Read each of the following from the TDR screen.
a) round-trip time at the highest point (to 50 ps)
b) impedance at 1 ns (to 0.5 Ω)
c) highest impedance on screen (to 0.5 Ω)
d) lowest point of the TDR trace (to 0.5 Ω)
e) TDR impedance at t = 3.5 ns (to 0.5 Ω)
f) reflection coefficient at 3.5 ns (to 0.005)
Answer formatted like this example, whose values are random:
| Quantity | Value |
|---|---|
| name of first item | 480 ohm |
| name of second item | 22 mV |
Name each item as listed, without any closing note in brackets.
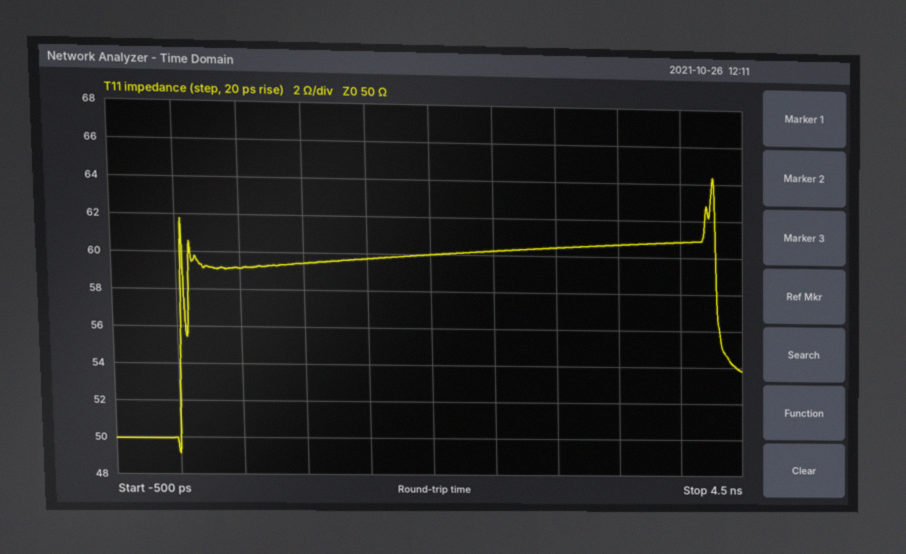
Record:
| Quantity | Value |
|---|---|
| round-trip time at the highest point | 4.25 ns |
| impedance at 1 ns | 59.5 Ω |
| highest impedance on screen | 64.5 Ω |
| lowest point of the TDR trace | 49.0 Ω |
| TDR impedance at t = 3.5 ns | 60.5 Ω |
| reflection coefficient at 3.5 ns | +0.095 |
